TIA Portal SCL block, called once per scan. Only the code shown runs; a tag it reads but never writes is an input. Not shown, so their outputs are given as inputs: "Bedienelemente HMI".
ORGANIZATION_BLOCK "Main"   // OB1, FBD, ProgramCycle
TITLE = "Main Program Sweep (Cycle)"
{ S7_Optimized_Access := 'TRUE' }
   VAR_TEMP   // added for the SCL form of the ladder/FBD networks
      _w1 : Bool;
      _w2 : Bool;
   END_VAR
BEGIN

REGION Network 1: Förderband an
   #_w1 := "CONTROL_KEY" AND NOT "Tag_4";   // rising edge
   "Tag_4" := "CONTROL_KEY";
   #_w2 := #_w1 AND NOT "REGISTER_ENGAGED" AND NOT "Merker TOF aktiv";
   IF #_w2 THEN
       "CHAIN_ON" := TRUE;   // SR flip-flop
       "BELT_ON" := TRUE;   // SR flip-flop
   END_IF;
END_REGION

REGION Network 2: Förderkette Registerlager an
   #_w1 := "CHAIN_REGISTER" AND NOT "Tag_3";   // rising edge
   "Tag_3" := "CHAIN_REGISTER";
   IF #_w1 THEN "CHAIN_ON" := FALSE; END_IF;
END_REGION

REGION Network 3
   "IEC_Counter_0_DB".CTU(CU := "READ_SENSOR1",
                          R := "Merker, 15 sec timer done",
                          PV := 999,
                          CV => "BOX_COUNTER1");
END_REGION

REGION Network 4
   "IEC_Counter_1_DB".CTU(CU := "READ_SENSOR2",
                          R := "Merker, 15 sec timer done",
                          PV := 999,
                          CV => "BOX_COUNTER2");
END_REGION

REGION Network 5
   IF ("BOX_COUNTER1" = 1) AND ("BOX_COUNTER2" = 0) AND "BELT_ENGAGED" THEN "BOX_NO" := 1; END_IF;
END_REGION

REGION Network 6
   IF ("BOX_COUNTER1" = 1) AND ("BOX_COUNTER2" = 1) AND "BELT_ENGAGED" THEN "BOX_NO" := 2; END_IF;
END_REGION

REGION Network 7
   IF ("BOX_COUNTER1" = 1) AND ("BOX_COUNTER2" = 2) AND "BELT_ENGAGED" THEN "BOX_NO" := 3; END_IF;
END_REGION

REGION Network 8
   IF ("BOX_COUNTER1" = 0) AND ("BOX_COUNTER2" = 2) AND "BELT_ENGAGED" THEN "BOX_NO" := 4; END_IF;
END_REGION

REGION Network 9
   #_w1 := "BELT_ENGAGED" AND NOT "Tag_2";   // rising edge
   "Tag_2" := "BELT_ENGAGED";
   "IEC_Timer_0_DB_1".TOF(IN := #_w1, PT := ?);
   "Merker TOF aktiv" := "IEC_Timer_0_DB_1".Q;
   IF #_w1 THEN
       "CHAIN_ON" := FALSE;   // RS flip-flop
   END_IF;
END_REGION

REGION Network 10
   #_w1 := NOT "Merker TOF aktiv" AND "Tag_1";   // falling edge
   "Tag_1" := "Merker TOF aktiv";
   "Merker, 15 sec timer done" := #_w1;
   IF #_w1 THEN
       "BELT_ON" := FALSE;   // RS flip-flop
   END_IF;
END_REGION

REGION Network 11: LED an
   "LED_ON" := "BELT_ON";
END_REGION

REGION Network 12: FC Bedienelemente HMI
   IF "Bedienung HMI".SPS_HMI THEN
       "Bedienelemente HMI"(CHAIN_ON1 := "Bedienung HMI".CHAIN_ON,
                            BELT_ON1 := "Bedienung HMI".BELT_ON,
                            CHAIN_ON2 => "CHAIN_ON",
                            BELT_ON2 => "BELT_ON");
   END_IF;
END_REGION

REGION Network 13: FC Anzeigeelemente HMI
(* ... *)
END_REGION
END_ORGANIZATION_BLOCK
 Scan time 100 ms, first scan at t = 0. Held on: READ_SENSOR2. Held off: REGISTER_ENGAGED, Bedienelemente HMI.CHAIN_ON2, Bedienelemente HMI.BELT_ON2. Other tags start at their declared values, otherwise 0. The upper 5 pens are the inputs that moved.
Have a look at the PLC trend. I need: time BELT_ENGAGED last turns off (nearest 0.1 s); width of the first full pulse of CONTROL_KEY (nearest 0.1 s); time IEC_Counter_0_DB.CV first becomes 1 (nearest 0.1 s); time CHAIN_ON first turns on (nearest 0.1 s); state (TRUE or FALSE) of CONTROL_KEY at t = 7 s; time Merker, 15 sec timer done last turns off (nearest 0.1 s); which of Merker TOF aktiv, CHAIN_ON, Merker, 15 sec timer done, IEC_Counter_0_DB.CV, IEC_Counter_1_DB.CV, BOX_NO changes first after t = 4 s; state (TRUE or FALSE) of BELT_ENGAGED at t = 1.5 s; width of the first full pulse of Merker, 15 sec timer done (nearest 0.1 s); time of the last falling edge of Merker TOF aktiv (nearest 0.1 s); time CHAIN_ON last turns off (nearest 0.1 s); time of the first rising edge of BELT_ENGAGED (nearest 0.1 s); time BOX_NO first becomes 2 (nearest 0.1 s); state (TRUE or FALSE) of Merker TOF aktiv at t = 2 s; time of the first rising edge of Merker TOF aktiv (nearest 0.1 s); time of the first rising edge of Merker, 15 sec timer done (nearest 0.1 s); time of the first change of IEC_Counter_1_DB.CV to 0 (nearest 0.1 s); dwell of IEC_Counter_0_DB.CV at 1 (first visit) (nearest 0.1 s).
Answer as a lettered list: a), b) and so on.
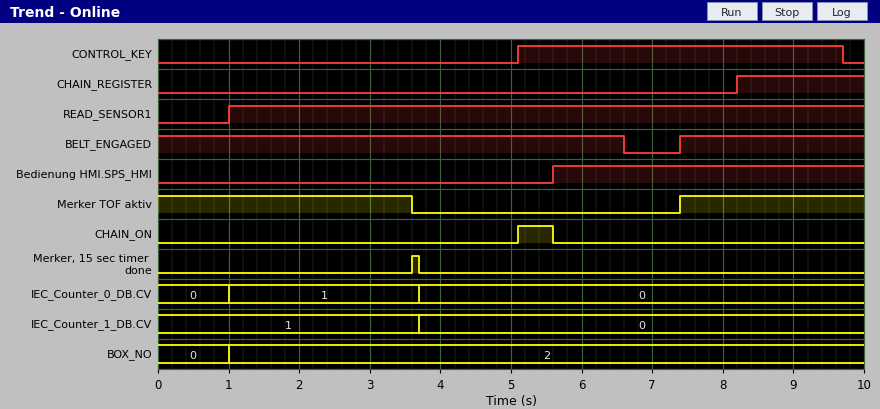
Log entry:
a) 6.6 s
b) 4.6 s
c) 1.0 s
d) 5.1 s
e) TRUE
f) 3.7 s
g) CHAIN_ON
h) TRUE
i) 0.1 s
j) 3.6 s
k) 5.6 s
l) 7.4 s
m) 1.0 s
n) TRUE
o) 7.4 s
p) 3.6 s
q) 3.7 s
r) 2.7 s
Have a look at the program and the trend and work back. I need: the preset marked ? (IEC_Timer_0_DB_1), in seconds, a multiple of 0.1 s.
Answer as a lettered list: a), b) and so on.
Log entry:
a) 3.5 s
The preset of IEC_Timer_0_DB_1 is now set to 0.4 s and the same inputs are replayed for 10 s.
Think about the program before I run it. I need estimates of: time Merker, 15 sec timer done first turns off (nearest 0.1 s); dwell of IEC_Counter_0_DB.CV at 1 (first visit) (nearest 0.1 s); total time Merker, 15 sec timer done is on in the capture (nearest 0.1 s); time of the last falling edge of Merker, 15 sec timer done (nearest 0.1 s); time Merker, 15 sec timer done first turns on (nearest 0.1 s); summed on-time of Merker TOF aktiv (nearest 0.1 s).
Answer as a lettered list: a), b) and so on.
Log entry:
a) 0.6 s
b) 7.0 s
c) 0.2 s
d) 8.0 s
e) 0.5 s
f) 1.0 s
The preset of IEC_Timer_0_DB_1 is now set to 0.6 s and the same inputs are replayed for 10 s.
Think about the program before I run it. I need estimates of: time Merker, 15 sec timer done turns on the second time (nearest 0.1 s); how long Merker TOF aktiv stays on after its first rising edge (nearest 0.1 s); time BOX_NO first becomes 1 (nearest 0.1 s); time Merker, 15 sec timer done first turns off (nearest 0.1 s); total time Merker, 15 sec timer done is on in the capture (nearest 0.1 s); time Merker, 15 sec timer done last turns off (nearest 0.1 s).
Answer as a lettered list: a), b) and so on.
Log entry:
a) 8.1 s
b) 0.7 s
c) 1.0 s
d) 0.8 s
e) 0.2 s
f) 8.2 s
